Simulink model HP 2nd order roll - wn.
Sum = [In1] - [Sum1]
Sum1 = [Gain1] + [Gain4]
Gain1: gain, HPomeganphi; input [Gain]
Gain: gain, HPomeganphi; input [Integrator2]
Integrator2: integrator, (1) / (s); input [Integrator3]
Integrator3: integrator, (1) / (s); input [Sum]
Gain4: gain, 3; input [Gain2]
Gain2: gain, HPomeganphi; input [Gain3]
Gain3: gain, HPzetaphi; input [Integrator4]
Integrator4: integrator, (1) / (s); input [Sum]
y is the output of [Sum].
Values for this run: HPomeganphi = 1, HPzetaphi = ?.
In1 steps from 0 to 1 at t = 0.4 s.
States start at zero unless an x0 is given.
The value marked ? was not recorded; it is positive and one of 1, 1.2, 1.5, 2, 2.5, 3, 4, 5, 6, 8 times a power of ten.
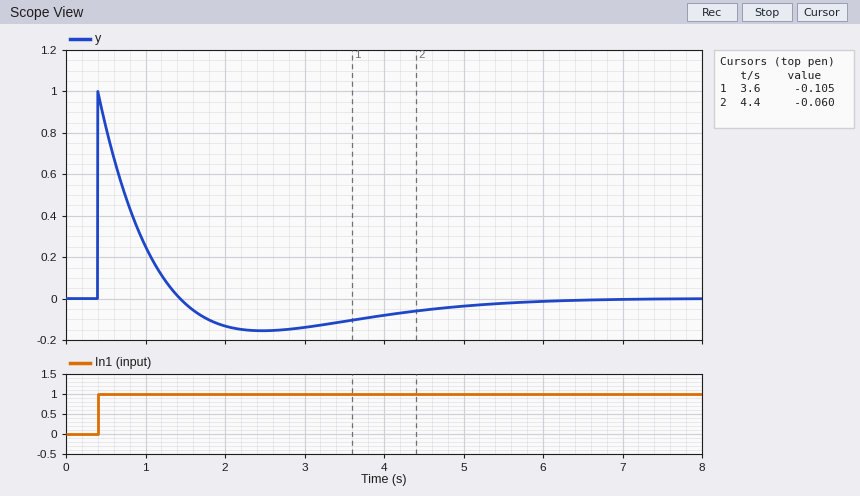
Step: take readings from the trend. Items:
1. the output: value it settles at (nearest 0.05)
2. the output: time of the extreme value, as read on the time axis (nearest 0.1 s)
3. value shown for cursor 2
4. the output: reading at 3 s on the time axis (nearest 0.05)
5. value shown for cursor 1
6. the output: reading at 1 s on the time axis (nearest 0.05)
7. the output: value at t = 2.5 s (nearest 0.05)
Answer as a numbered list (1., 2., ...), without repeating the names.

1. 0.00
2. 0.4 s
3. -0.060
4. -0.15
5. -0.105
6. 0.25
7. -0.15
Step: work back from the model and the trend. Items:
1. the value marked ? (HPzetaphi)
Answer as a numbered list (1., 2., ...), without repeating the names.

1. 0.6
